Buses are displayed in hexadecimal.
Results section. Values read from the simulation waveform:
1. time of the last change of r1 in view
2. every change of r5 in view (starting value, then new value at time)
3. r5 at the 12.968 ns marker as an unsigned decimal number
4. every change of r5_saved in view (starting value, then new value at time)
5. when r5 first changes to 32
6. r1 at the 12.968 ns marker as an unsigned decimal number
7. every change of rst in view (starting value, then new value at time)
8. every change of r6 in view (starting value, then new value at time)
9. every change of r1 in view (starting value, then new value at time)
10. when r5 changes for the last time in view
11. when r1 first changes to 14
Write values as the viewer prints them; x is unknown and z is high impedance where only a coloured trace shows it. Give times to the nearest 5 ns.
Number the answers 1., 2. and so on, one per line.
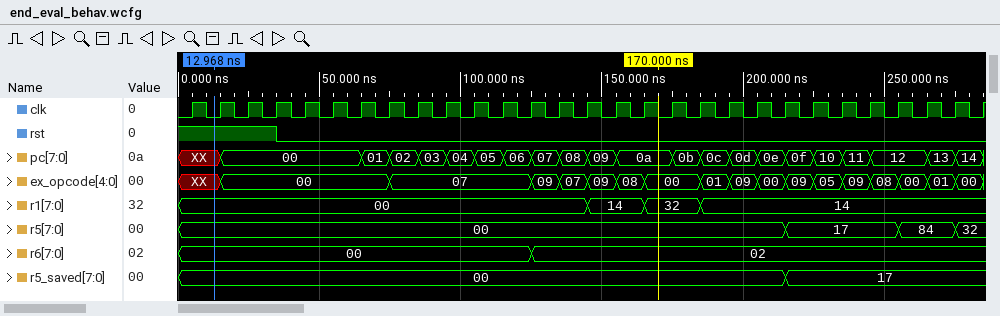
1. 185 ns
2. 00, 17 at 215 ns, 84 at 255 ns, 32 at 275 ns
3. 0
4. 00, 17 at 215 ns
5. 275 ns
6. 0
7. 1, 0 at 35 ns
8. 00, 02 at 125 ns
9. 00, 14 at 145 ns, 32 at 165 ns, 14 at 185 ns
10. 275 ns
11. 145 ns
